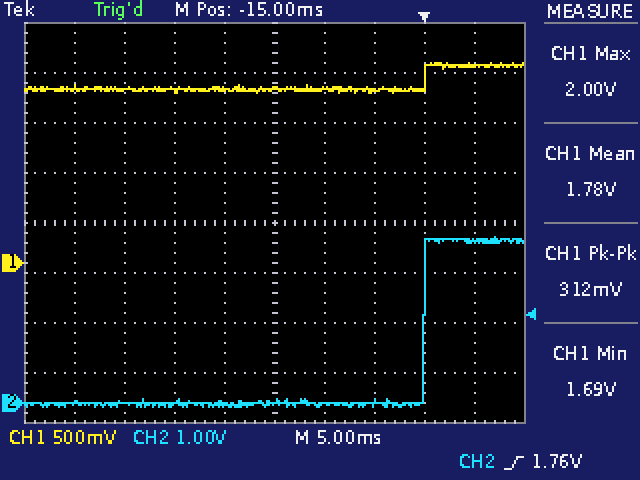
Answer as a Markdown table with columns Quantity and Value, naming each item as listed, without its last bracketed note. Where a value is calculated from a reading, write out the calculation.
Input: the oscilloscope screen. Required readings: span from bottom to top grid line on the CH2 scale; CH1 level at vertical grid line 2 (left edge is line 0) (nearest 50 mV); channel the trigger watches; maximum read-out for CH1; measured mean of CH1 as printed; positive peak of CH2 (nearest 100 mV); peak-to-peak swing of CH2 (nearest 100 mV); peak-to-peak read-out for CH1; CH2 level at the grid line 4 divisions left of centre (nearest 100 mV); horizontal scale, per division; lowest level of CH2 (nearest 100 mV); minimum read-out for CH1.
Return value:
| Quantity | Value |
|---|---|
| span from bottom to top grid line on the CH2 scale | 8 V |
| CH1 level at vertical grid line 2 (left edge is line 0) | 1.75 V |
| channel the trigger watches | CH2 |
| maximum read-out for CH1 | 2.00 V |
| measured mean of CH1 as printed | 1.78 V |
| positive peak of CH2 | 3.3 V |
| peak-to-peak swing of CH2 | 3.3 V − (-100 mV) = 3.4 V |
| peak-to-peak read-out for CH1 | 312 mV |
| CH2 level at the grid line 4 divisions left of centre | 0.0 V |
| horizontal scale, per division | 5 ms |
| lowest level of CH2 | -100 mV |
| minimum read-out for CH1 | 1.69 V |
